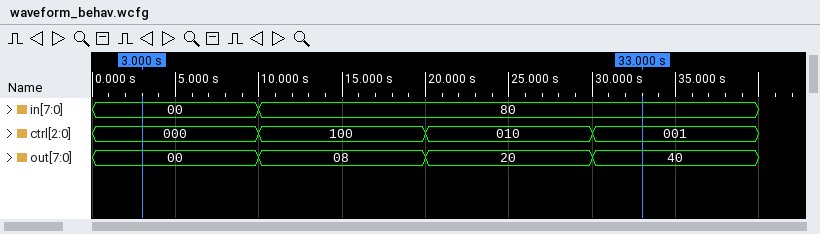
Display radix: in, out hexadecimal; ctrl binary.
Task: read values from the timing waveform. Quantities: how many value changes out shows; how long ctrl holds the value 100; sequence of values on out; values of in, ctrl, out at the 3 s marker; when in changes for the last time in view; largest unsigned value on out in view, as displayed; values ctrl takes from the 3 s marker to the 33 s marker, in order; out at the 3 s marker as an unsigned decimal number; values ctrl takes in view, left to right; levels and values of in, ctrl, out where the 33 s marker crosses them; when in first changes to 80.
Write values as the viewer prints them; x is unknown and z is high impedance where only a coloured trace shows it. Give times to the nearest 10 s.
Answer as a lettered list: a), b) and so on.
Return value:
a) 3
b) 10 s
c) 00, 08, 20, 40
d) in=00, ctrl=000, out=00
e) 10 s
f) 40
g) 000, 100, 010, 001
h) 0
i) 000, 100, 010, 001
j) in=80, ctrl=001, out=40
k) 10 s
